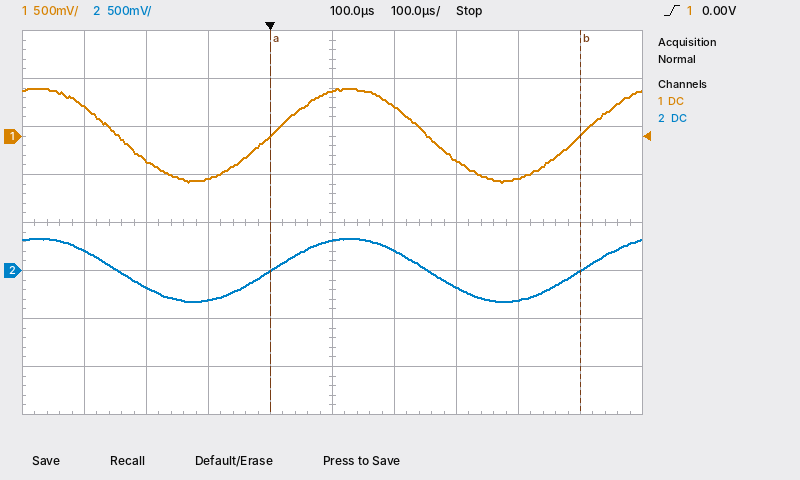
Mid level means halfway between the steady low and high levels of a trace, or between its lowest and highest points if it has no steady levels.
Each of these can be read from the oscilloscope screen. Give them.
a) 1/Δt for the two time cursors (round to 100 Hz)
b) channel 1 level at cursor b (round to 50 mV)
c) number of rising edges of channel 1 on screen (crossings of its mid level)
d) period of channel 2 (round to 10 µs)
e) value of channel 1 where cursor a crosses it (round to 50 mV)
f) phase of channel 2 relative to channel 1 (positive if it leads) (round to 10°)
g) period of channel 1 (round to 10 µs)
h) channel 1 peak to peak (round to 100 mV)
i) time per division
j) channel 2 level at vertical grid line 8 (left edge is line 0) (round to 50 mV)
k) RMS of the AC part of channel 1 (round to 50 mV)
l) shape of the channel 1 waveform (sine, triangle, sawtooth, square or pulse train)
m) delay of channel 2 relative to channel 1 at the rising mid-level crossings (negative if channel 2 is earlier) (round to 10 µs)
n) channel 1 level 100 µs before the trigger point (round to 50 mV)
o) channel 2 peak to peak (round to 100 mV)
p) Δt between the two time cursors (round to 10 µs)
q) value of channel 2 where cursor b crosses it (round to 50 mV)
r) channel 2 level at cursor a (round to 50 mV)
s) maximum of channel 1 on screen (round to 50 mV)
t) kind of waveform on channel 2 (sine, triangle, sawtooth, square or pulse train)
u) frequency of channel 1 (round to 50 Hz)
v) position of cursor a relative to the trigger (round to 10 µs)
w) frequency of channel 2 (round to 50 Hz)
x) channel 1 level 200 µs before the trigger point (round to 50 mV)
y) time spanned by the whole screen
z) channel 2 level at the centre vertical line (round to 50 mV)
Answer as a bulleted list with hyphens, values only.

- 2.0 kHz
- 0 mV
- 2
- 500 µs
- 0 mV
- 0°
- 500 µs
- 1.00 V
- 100 µs
- -300 mV
- 350 mV
- sine
- 0 µs
- -450 mV
- 700 mV
- 500 µs
- 0 mV
- 0 mV
- 500 mV
- sine
- 2.00 kHz
- 0 µs
- 2.00 kHz
- -250 mV
- 1 ms
- 300 mV
